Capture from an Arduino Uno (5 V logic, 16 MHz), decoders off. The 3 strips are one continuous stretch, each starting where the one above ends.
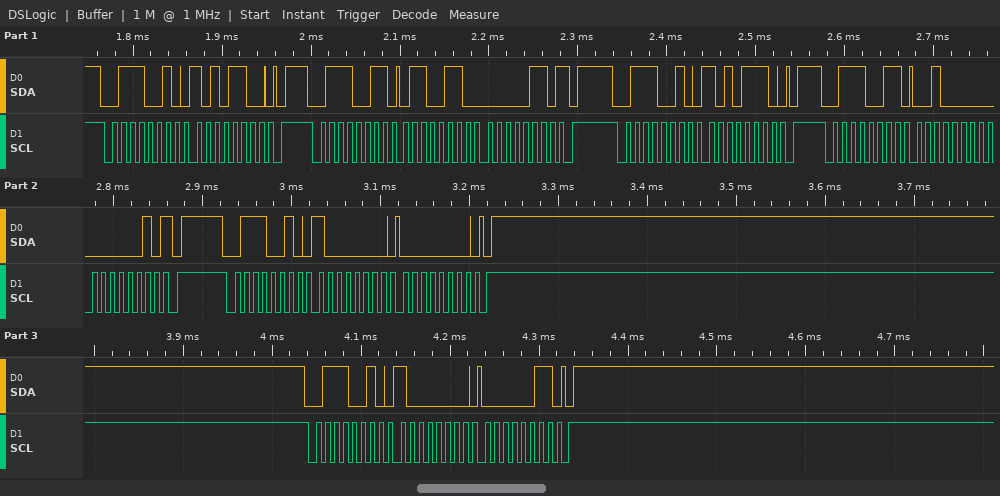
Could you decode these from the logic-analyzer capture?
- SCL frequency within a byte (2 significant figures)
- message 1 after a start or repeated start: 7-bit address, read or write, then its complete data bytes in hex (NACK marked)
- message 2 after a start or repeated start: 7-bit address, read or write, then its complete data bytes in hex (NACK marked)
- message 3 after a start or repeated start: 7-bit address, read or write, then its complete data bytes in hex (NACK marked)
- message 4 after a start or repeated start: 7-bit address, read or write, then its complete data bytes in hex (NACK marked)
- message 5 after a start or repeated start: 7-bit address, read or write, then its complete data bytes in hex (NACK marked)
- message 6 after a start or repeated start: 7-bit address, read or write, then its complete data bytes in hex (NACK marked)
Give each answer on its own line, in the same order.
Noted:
100 kHz
0x39 write: AC
0x39 read: 66 06 NACK
0x39 write: AE
0x39 read: 20 02 NACK
0x39 write: 80 00
0x39 write: 80 03
